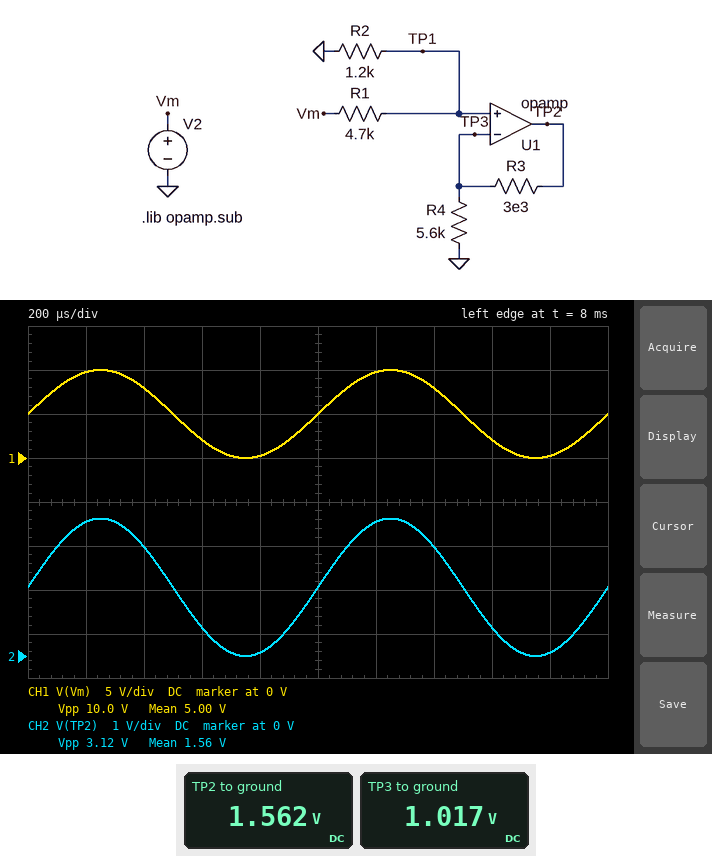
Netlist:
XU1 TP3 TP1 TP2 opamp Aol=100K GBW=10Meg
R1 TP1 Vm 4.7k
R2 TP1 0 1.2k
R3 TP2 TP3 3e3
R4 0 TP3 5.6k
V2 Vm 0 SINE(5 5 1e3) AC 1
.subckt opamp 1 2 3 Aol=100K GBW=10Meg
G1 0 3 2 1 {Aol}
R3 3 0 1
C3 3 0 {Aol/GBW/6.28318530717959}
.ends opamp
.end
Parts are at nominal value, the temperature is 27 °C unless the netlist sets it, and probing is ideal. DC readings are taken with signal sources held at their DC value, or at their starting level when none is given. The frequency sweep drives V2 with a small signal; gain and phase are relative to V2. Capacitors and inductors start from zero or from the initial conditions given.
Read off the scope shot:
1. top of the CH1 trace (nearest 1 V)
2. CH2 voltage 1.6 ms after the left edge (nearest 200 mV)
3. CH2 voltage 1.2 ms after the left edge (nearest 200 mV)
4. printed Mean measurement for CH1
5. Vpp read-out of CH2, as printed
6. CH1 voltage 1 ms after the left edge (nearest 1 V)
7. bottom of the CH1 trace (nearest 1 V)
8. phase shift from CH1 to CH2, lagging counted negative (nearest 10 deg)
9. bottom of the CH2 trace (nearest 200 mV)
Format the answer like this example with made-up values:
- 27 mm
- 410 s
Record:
- 10 V
- 600 mV
- 3.0 V
- 5.00 V
- 3.12 V
- 5 V
- 0 V
- 0 deg
- 0 V
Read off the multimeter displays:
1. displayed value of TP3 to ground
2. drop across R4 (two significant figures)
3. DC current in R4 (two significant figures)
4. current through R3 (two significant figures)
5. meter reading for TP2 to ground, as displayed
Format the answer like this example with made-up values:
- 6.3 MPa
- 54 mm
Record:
- 1.017 V
- 1.0 V
- 180 µA
- 180 µA
- 1.562 V
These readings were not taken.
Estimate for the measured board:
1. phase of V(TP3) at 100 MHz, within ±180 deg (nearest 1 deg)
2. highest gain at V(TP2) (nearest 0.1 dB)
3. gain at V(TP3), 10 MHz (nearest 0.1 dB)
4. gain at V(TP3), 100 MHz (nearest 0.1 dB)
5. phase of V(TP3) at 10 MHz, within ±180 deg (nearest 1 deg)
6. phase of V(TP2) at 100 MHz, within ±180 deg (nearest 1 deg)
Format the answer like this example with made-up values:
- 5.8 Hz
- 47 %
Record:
- -86 deg
- -10.1 dB
- -19.1 dB
- -37.6 dB
- -57 deg
- -86 deg
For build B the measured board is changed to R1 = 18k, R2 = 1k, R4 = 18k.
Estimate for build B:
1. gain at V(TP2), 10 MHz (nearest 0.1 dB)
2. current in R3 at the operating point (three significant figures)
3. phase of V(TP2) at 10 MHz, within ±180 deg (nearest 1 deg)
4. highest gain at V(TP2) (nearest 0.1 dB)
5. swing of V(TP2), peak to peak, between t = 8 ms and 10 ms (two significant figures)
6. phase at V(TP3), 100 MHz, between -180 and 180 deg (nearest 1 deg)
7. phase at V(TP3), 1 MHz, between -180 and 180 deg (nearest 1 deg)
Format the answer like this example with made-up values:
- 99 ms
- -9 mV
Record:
- -28.0 dB
- 14.6 µA
- -49 deg
- -24.2 dB
- 610 mV
- -85 deg
- -7 deg
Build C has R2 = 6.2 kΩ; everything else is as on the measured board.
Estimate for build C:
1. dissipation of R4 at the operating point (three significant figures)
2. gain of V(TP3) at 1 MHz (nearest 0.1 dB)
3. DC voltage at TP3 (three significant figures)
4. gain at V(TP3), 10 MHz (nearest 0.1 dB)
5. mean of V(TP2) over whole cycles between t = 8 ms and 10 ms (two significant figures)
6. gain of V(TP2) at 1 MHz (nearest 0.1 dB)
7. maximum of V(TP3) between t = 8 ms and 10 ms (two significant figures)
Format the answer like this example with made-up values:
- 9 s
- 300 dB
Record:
- 1.44 mW
- -5.0 dB
- 2.84 V
- -10.2 dB
- 4.4 V
- -1.3 dB
- 5.7 V
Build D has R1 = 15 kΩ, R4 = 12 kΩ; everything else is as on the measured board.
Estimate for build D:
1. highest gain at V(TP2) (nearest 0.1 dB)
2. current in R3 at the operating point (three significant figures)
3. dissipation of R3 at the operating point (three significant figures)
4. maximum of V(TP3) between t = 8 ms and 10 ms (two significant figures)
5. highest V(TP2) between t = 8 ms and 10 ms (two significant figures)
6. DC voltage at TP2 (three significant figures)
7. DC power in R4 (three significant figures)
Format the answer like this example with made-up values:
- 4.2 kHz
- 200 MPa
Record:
- -20.7 dB
- 30.9 µA
- 2.86 µW
- 740 mV
- 930 mV
- 463 mV
- 11.4 µW
